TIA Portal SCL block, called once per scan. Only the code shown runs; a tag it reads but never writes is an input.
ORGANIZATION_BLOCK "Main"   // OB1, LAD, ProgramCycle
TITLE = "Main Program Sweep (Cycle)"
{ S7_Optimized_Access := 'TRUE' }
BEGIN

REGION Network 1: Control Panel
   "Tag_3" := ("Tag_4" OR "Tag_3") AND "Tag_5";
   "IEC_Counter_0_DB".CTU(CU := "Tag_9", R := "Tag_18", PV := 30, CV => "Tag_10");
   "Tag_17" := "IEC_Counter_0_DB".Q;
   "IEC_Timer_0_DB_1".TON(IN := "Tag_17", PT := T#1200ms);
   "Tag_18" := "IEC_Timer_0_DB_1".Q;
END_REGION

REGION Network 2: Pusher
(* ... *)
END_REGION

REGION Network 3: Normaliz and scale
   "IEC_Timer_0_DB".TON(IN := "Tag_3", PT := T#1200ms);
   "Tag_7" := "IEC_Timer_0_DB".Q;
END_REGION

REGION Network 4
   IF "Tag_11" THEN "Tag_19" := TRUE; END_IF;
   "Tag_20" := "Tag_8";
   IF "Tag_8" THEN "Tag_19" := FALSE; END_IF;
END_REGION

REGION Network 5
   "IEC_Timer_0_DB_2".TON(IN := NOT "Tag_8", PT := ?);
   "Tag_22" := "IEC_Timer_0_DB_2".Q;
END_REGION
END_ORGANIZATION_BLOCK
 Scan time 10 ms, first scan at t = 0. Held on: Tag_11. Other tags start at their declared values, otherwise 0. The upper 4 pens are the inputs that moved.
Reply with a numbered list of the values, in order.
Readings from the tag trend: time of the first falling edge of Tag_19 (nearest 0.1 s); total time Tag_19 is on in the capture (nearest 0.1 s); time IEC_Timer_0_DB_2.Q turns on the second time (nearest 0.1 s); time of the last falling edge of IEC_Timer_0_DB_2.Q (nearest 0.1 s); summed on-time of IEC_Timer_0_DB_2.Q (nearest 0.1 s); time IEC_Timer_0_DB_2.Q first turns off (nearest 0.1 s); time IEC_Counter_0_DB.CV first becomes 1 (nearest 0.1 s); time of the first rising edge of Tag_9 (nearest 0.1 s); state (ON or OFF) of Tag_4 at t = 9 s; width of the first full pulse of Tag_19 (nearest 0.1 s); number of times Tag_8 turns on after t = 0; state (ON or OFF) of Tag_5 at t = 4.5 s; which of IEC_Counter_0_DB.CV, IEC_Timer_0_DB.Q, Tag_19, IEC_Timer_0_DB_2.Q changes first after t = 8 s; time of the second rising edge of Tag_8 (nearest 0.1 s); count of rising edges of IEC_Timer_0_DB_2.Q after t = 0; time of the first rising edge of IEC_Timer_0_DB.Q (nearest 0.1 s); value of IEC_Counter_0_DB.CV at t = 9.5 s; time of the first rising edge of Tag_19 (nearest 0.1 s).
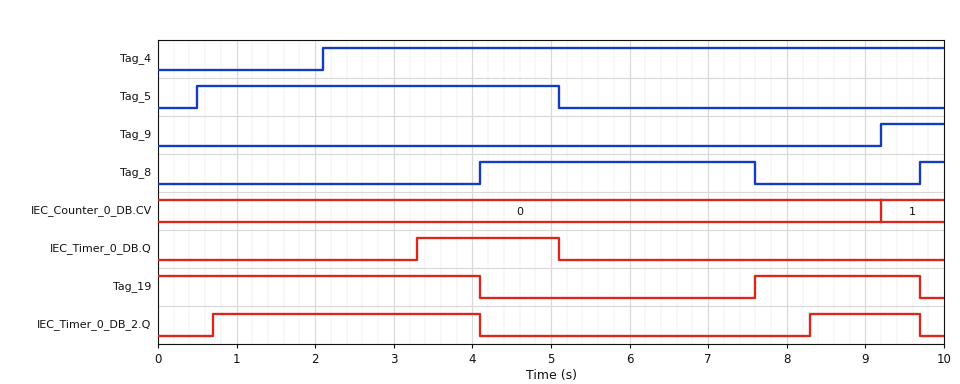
1. 4.1 s
2. 6.2 s
3. 8.3 s
4. 9.7 s
5. 4.8 s
6. 4.1 s
7. 9.2 s
8. 9.2 s
9. ON
10. 2.1 s
11. 2
12. ON
13. IEC_Timer_0_DB_2.Q
14. 9.7 s
15. 2
16. 3.3 s
17. 1
18. 7.6 s
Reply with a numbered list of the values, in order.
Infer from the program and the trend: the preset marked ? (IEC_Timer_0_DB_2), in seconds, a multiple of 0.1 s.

1. 0.7 s
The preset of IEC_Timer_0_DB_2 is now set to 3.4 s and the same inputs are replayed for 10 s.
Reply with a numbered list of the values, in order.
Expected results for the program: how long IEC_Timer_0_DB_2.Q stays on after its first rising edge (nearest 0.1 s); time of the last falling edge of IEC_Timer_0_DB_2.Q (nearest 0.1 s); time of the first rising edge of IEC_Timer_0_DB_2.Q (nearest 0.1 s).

1. 0.7 s
2. 4.1 s
3. 3.4 s
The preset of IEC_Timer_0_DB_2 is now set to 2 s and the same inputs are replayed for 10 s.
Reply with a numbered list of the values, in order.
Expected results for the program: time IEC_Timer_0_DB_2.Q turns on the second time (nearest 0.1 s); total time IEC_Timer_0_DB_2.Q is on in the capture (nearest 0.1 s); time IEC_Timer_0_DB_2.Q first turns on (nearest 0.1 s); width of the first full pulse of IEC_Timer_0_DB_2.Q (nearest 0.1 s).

1. 9.6 s
2. 2.2 s
3. 2.0 s
4. 2.1 s
